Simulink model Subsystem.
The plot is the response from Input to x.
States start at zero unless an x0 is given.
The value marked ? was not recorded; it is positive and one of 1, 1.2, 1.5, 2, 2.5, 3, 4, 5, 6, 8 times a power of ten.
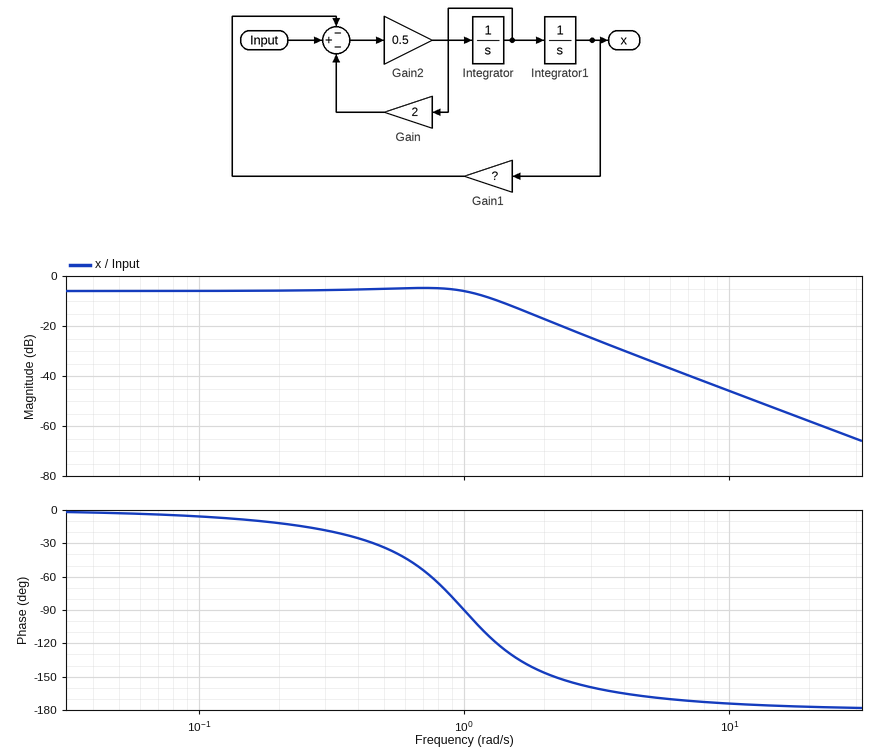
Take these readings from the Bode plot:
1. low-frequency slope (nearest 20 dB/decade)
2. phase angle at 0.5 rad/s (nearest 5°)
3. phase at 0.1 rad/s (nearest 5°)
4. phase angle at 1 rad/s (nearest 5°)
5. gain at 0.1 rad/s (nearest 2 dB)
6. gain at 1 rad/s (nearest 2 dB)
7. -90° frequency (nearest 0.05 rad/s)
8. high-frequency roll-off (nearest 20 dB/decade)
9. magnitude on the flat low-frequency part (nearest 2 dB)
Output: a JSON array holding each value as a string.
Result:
["0 dB/decade", "-35°", "-5°", "-90°", "-6 dB", "-6 dB", "1.00 rad/s", "-40 dB/decade", "-6 dB"]
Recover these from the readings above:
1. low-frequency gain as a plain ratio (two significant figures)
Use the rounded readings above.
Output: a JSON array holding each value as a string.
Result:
["0.50"]
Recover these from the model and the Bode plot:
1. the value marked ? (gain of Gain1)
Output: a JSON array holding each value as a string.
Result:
["2"]
